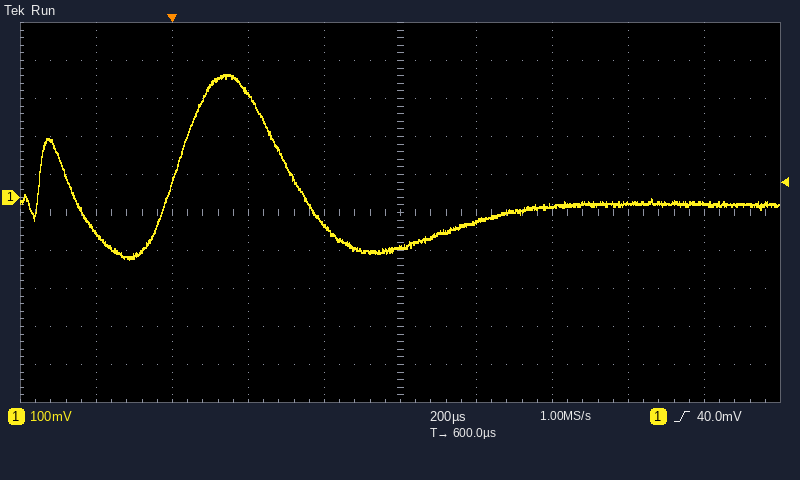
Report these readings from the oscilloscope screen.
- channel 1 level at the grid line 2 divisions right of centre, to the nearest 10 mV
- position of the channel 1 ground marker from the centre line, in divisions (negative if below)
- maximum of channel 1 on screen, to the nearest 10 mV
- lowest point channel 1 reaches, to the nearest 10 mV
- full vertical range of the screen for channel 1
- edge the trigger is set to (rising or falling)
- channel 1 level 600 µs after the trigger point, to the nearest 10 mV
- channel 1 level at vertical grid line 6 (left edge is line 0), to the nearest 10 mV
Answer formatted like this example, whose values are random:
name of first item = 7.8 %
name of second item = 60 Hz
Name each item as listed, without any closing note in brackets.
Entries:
channel 1 level at the grid line 2 divisions right of centre, to the nearest 10 mV = -20 mV
position of the channel 1 ground marker from the centre line, in divisions = +0.4 div
maximum of channel 1 on screen, to the nearest 10 mV = 320 mV
lowest point channel 1 reaches, to the nearest 10 mV = -160 mV
full vertical range of the screen for channel 1 = 1 V
edge the trigger is set to = rising
channel 1 level 600 µs after the trigger point, to the nearest 10 mV = -130 mV
channel 1 level at vertical grid line 6 (left edge is line 0), to the nearest 10 mV = -60 mV
